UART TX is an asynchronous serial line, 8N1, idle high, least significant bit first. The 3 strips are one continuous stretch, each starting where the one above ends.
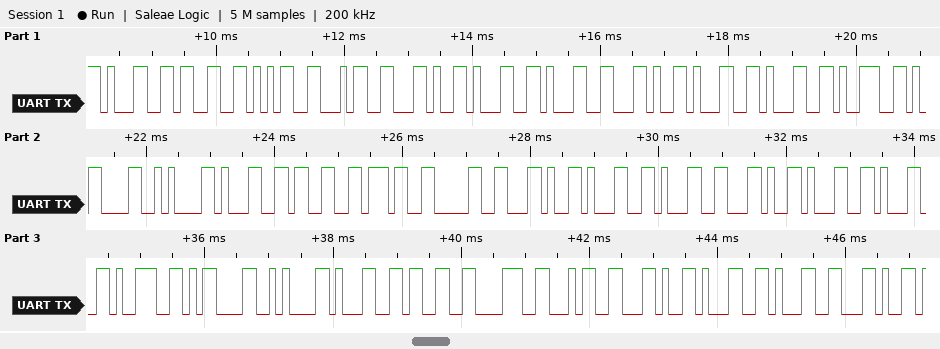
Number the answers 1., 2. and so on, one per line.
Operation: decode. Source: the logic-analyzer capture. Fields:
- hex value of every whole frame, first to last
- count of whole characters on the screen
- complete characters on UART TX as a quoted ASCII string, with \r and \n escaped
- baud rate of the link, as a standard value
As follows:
1. 31 33 35 34 2C 31 31 2C 31 31 39 0D 0A 31 33 37 30 2C 31 31 2C 31 31 39 0D 0A 31 33 38 34 2C 31 31 2C
2. 34
3. "1354,11,119\r\n1370,11,119\r\n1384,11,"
4. 9600 baud
